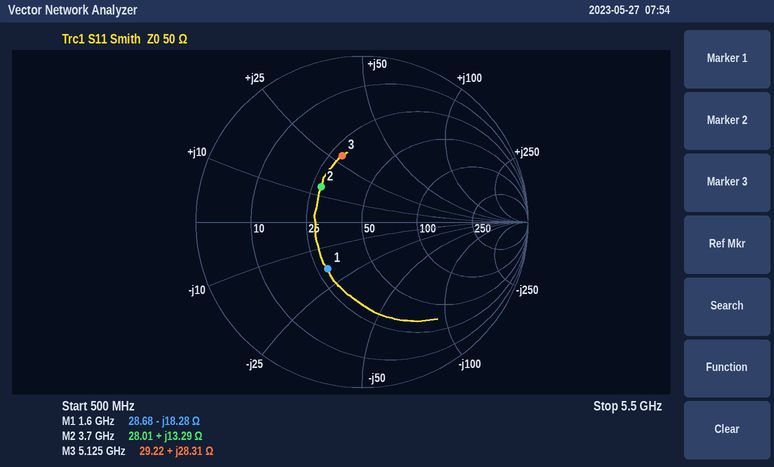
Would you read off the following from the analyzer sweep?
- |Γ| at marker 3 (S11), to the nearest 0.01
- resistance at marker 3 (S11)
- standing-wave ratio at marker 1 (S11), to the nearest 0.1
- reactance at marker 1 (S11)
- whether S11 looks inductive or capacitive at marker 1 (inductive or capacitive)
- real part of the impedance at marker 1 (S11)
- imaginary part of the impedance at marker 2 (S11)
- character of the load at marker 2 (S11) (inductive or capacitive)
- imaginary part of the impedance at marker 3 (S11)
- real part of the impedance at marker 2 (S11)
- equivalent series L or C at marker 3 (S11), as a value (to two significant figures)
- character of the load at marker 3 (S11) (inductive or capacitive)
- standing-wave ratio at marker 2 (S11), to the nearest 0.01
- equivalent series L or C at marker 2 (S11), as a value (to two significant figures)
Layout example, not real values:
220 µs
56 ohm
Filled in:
0.42
29.22 Ω
2.1
-18.28 Ω
capacitive
28.68 Ω
+13.29 Ω
inductive
+28.31 Ω
28.01 Ω
880 pH
inductive
1.96
570 pH
